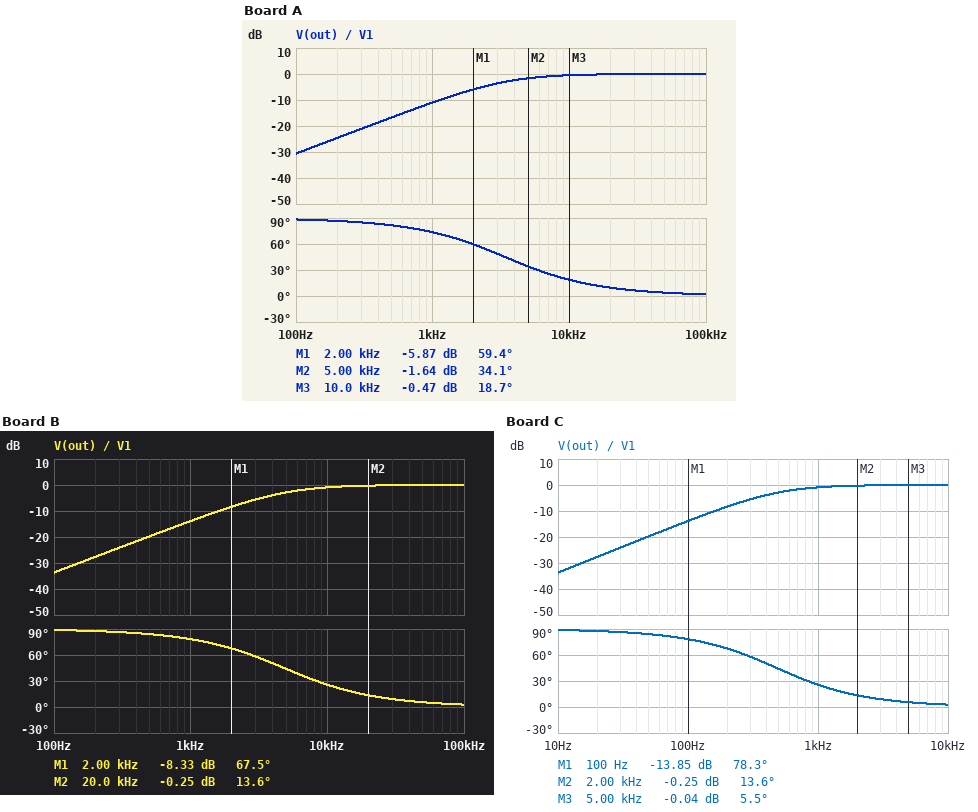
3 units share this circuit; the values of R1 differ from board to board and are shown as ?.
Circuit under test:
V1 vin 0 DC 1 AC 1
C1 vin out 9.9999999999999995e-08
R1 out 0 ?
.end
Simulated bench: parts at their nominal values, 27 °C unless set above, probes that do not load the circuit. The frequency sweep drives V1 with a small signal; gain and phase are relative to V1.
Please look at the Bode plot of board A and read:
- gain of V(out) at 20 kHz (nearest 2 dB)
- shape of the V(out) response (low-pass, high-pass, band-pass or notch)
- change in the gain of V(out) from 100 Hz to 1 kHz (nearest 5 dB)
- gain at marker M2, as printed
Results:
0 dB
high-pass
20 dB
-1.64 dB
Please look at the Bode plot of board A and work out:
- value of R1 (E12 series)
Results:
470 Ω
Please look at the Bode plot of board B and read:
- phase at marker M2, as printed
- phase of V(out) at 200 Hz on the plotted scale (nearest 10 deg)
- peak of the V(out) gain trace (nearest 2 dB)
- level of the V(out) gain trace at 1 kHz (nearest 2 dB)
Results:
13.6 deg
90 deg
0 dB
-14 dB
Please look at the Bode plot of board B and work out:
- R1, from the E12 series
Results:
330 Ω
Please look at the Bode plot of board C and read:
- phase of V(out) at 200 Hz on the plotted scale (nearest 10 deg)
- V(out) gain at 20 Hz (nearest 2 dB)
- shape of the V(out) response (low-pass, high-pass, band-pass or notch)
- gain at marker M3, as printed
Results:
70 deg
-28 dB
high-pass
-0.04 dB
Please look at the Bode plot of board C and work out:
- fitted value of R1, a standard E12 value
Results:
3.3 kΩ
